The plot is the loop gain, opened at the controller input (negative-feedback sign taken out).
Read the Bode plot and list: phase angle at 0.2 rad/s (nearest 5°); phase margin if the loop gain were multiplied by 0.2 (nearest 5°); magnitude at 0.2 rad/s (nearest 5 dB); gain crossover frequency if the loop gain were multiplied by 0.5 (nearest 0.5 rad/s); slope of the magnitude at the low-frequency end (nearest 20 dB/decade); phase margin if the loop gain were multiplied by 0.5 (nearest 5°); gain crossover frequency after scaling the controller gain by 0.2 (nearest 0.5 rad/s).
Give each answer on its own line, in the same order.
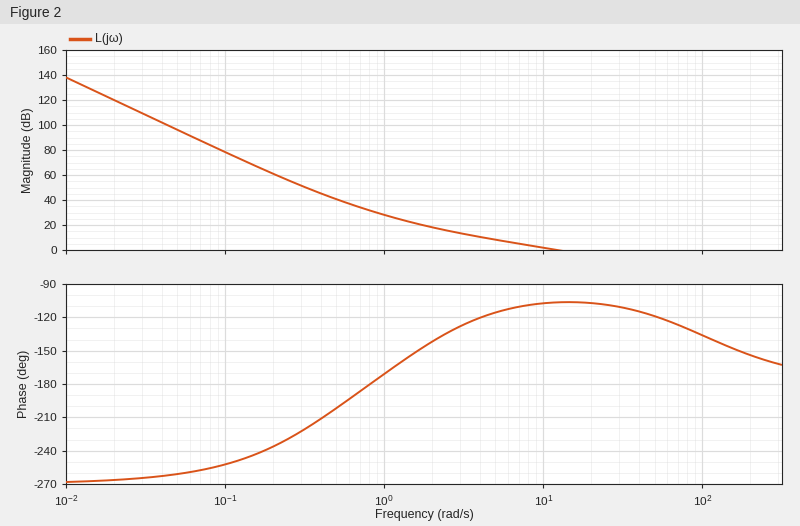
-235°
50°
60 dB
6.5 rad/s
-60 dB/decade
70°
3.0 rad/s
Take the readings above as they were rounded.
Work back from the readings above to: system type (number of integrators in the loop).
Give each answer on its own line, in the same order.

3
